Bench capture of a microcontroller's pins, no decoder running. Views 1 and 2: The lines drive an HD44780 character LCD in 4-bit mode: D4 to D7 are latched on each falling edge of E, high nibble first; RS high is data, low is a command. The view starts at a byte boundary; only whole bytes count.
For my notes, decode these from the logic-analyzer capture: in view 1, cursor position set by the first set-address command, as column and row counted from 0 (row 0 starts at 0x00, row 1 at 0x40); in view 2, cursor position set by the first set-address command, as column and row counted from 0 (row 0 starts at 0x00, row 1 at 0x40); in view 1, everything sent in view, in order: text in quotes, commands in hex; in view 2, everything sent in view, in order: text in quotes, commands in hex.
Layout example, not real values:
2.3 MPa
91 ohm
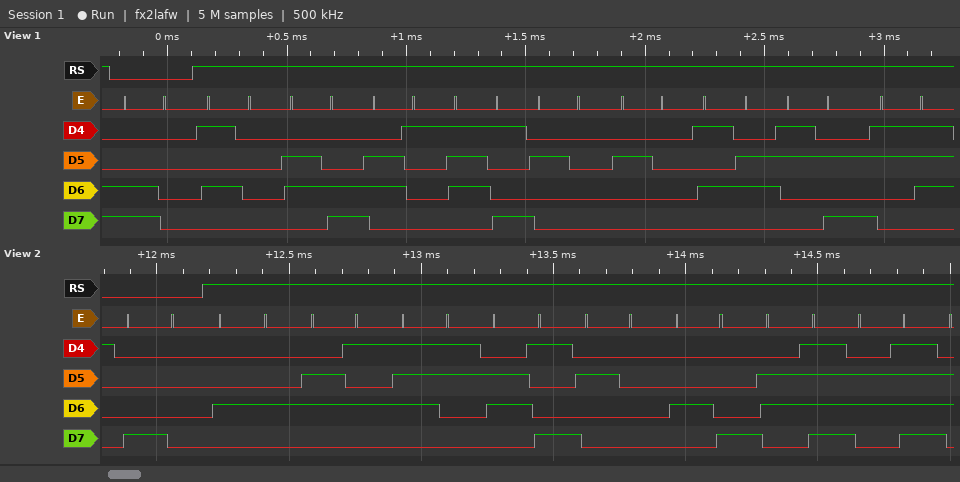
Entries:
column 0, row 1
column 0, row 0
0xC0 "Play  V:7"
0x80 "Desi Hoo"
